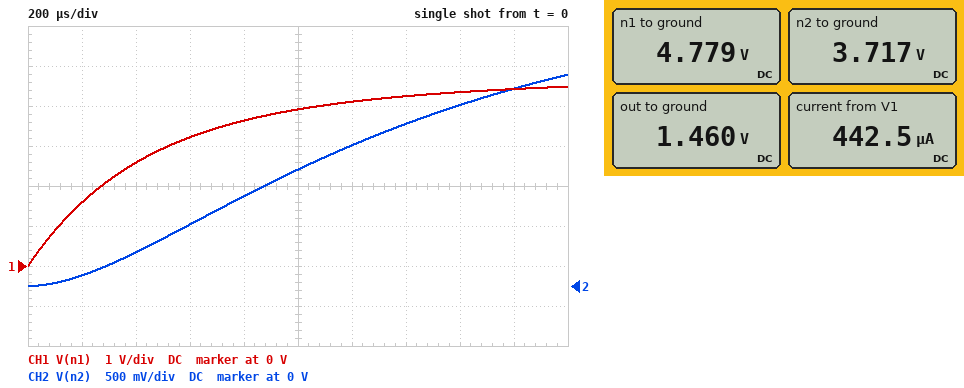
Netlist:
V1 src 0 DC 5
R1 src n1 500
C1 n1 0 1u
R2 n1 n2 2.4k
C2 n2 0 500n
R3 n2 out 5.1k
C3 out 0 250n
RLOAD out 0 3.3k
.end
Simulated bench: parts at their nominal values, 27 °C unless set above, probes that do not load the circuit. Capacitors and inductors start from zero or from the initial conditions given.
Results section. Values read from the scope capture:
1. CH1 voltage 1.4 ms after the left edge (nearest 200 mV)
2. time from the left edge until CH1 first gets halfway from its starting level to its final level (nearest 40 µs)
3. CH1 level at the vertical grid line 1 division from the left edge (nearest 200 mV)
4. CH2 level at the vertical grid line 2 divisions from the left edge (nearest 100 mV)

4.2 V
320 µs
1.6 V
400 mV
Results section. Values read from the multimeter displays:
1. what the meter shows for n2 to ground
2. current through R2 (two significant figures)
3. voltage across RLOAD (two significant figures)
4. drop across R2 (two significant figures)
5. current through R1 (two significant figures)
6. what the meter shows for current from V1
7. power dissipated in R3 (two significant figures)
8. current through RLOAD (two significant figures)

3.717 V
440 µA
1.5 V
1.1 V
440 µA
442.5 µA
1.0 mW
440 µA
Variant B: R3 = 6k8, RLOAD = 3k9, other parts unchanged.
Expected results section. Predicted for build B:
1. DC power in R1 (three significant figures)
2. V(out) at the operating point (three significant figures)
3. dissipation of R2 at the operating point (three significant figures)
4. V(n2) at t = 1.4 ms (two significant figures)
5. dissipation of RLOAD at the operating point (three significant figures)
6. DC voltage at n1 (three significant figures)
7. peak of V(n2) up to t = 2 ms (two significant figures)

67.6 µW
1.43 V
324 µW
2.1 V
527 µW
4.82 V
2.7 V
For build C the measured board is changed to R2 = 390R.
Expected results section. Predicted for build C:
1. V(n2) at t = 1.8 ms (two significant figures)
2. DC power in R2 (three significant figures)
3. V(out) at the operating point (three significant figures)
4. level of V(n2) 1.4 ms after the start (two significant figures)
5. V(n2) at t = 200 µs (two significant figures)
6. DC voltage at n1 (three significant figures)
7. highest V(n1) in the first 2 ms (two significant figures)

4.0 V
113 µW
1.78 V
3.6 V
560 mV
4.73 V
4.4 V
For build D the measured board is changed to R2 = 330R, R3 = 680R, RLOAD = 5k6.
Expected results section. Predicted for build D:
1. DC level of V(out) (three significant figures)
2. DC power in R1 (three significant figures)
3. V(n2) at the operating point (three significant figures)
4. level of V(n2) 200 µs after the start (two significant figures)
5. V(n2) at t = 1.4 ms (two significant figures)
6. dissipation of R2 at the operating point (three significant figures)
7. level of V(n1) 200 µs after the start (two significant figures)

3.94 V
247 µW
4.42 V
560 mV
3.4 V
163 µW
1.4 V
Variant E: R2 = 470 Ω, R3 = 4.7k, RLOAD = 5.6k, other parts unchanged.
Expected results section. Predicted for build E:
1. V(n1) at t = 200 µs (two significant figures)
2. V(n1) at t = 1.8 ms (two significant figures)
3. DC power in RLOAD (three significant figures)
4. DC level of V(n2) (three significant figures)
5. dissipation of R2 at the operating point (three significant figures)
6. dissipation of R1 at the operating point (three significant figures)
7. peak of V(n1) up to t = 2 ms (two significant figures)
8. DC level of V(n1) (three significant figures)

1.4 V
4.3 V
1.10 mW
4.57 V
92.5 µW
98.4 µW
4.4 V
4.78 V
